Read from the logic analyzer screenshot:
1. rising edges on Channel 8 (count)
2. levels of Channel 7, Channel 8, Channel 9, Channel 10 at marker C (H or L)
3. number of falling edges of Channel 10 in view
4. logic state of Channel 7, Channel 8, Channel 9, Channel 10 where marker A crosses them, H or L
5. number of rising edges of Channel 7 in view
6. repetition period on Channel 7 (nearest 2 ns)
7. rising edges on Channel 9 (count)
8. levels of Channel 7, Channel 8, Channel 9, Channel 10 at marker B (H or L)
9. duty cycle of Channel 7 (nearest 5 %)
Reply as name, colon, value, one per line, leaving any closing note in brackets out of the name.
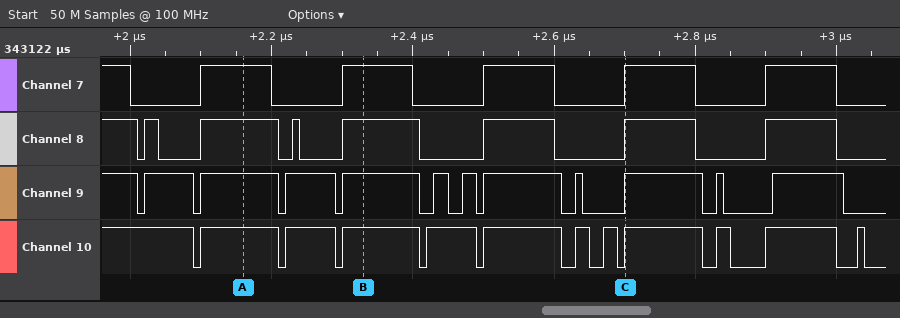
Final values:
rising edges on Channel 8: 7
levels of Channel 7, Channel 8, Channel 9, Channel 10 at marker C: Channel 7=H, Channel 8=H, Channel 9=H, Channel 10=H
number of falling edges of Channel 10 in view: 12
logic state of Channel 7, Channel 8, Channel 9, Channel 10 where marker A crosses them, H or L: Channel 7=H, Channel 8=H, Channel 9=H, Channel 10=H
number of rising edges of Channel 7 in view: 5
repetition period on Channel 7: 200 ns
rising edges on Channel 9: 11
levels of Channel 7, Channel 8, Channel 9, Channel 10 at marker B: Channel 7=H, Channel 8=H, Channel 9=H, Channel 10=H
duty cycle of Channel 7: 50 %
